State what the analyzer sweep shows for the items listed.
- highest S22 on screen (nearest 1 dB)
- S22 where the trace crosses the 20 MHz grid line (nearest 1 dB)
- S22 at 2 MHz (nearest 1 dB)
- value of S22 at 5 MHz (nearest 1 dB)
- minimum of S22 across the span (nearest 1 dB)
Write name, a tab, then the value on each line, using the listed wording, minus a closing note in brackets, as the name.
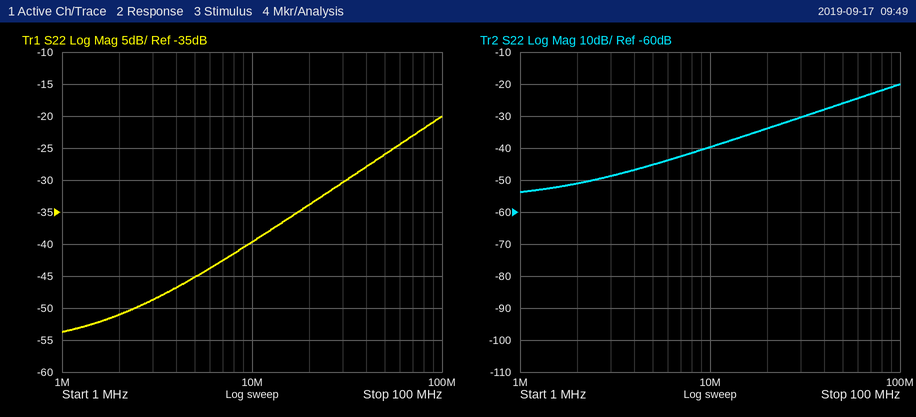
highest S22 on screen	-20 dB
S22 where the trace crosses the 20 MHz grid line	-34 dB
S22 at 2 MHz	-51 dB
value of S22 at 5 MHz	-45 dB
minimum of S22 across the span	-54 dB
